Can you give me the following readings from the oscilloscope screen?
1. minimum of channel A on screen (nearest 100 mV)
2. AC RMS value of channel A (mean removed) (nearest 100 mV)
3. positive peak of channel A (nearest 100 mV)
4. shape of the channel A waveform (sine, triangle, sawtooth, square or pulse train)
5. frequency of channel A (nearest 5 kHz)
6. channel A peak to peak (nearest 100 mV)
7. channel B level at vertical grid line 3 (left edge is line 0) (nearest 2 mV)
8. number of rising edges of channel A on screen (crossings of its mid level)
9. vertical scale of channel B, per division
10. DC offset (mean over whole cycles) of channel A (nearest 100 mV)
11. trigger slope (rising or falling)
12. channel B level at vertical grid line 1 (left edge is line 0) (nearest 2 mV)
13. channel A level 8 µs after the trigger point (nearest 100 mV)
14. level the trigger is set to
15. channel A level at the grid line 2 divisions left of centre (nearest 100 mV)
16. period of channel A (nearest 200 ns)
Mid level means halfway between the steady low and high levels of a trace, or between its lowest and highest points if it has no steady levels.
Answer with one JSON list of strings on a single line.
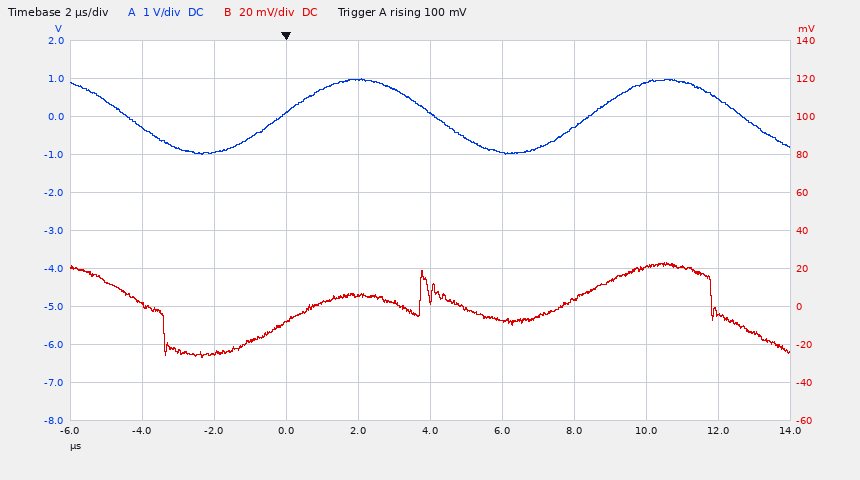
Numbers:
["-1.0 V", "700 mV", "1.0 V", "sine", "115 kHz", "2.0 V", "-8 mV", "2", "20 mV", "0.0 V", "rising", "0 mV", "-300 mV", "100 mV", "100 mV", "8.6 µs"]
